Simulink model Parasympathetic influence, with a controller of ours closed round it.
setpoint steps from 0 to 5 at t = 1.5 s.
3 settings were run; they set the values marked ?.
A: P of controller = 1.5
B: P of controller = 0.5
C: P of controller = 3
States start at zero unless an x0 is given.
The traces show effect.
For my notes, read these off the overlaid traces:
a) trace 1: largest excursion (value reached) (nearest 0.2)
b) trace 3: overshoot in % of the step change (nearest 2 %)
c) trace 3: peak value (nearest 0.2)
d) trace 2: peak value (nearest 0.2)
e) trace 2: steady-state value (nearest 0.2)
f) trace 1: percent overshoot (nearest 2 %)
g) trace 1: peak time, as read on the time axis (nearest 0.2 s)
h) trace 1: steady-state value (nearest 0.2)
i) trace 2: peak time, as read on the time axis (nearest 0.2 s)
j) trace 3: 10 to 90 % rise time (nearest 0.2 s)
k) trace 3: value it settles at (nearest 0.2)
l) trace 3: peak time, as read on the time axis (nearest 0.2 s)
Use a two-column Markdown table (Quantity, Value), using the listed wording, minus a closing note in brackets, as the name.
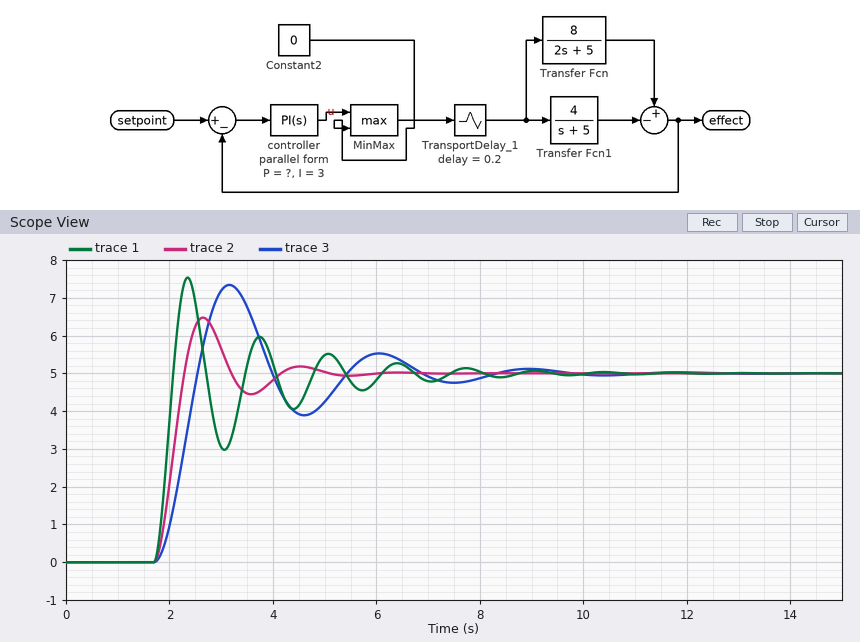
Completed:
| Quantity | Value |
|---|---|
| trace 1: largest excursion (value reached) | 7.6 |
| trace 3: overshoot in % of the step change | 46 % |
| trace 3: peak value | 7.4 |
| trace 2: peak value | 6.4 |
| trace 2: steady-state value | 5.0 |
| trace 1: percent overshoot | 50 % |
| trace 1: peak time, as read on the time axis | 2.4 s |
| trace 1: steady-state value | 5.0 |
| trace 2: peak time, as read on the time axis | 2.6 s |
| trace 3: 10 to 90 % rise time | 0.6 s |
| trace 3: value it settles at | 5.0 |
| trace 3: peak time, as read on the time axis | 3.2 s |
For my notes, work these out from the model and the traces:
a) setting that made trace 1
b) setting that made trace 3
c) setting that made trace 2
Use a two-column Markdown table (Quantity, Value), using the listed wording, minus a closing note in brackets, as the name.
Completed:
| Quantity | Value |
|---|---|
| setting that made trace 1 | C |
| setting that made trace 3 | B |
| setting that made trace 2 | A |
